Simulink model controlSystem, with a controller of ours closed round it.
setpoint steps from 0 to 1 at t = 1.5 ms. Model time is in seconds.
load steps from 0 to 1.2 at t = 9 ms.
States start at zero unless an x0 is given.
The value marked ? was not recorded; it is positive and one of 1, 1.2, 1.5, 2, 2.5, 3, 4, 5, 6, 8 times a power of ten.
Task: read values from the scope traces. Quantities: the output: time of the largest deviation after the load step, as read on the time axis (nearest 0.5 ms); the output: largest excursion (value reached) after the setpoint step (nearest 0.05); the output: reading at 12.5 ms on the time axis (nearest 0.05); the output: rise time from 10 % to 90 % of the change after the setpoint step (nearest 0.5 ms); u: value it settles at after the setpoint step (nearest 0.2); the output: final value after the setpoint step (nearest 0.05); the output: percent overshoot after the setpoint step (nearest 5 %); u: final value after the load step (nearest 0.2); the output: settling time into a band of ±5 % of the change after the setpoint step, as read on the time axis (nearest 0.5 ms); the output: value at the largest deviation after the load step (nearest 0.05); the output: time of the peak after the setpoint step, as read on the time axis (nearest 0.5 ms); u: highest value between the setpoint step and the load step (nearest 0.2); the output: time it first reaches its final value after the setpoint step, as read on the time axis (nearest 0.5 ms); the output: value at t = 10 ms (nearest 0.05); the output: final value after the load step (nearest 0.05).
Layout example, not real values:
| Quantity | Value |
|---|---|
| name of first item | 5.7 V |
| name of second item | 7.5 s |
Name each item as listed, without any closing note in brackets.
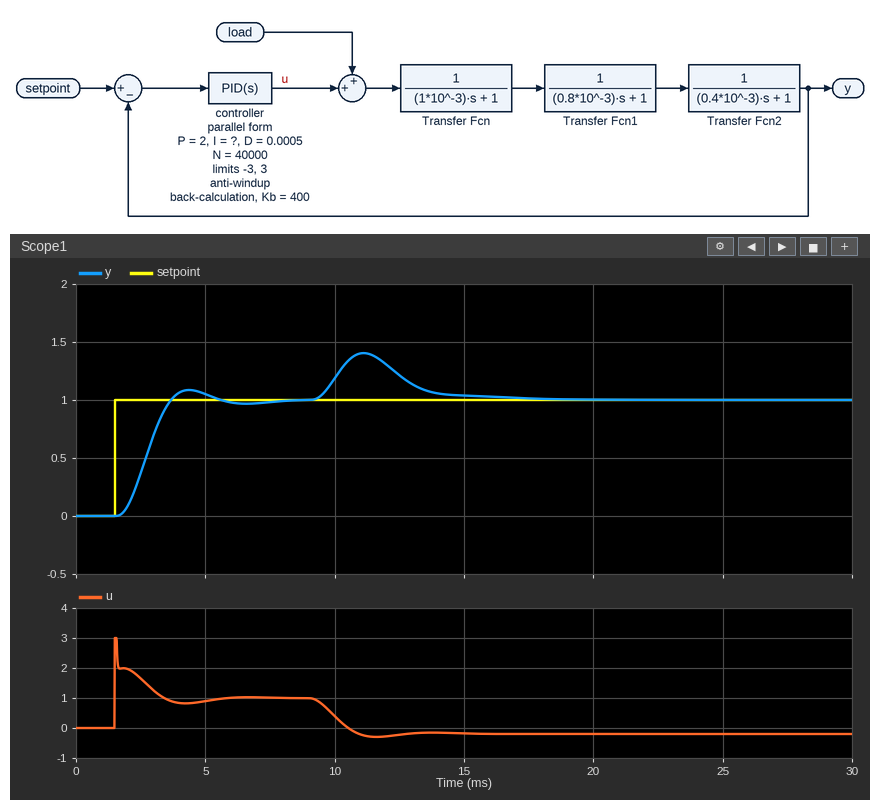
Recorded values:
| Quantity | Value |
|---|---|
| the output: time of the largest deviation after the load step, as read on the time axis | 11.0 ms |
| the output: largest excursion (value reached) after the setpoint step | 1.10 |
| the output: reading at 12.5 ms on the time axis | 1.20 |
| the output: rise time from 10 % to 90 % of the change after the setpoint step | 1.5 ms |
| u: value it settles at after the setpoint step | 1.0 |
| the output: final value after the setpoint step | 1.00 |
| the output: percent overshoot after the setpoint step | 10 % |
| u: final value after the load step | -0.2 |
| the output: settling time into a band of ±5 % of the change after the setpoint step, as read on the time axis | 5.0 ms |
| the output: value at the largest deviation after the load step | 1.40 |
| the output: time of the peak after the setpoint step, as read on the time axis | 4.5 ms |
| u: highest value between the setpoint step and the load step | 3.0 |
| the output: time it first reaches its final value after the setpoint step, as read on the time axis | 3.5 ms |
| the output: value at t = 10 ms | 1.20 |
| the output: final value after the load step | 1.00 |
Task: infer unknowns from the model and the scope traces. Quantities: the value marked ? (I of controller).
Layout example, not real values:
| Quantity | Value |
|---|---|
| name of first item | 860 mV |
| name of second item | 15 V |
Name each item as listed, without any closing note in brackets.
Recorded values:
| Quantity | Value |
|---|---|
| the value marked ? | 1000 |
